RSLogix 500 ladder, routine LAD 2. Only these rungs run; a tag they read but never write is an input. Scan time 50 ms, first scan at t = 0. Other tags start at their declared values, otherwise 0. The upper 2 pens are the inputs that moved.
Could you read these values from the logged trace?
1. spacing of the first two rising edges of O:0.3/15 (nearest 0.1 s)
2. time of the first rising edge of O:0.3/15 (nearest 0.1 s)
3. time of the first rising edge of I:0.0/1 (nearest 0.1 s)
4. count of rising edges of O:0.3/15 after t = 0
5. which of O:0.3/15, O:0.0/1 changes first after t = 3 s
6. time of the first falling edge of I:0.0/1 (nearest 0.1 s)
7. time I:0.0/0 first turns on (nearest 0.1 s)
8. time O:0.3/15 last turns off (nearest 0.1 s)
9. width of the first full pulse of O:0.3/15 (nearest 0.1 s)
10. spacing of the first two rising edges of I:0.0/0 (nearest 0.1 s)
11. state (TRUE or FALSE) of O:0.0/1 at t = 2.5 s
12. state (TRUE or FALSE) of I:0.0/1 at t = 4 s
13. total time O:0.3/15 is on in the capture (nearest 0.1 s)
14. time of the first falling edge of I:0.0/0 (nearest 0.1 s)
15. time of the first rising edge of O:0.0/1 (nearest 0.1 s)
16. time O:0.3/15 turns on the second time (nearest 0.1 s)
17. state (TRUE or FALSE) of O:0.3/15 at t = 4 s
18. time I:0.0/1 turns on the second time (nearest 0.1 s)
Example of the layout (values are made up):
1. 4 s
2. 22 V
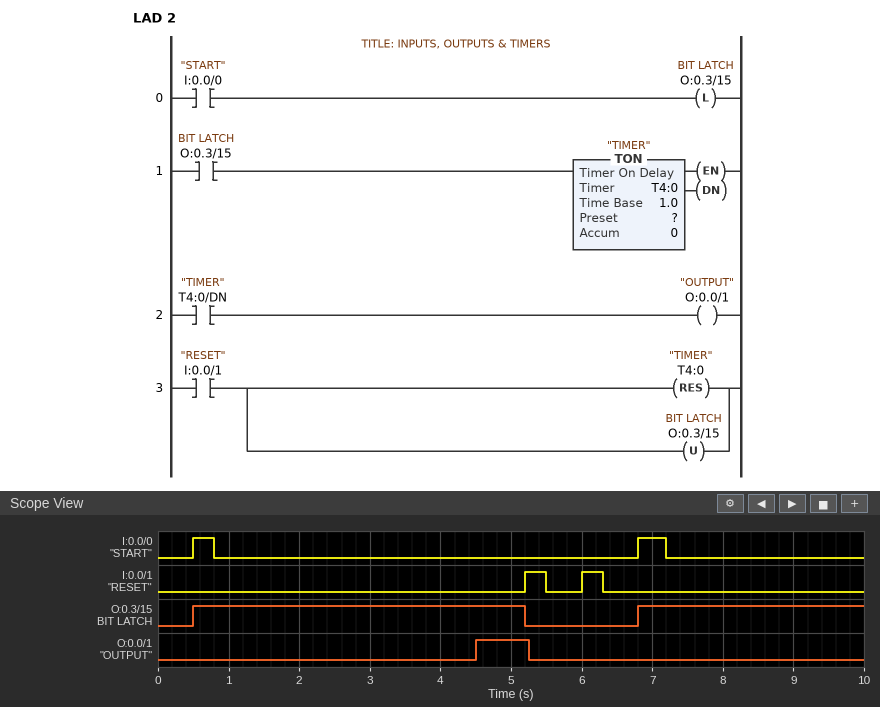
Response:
1. 6.3 s
2. 0.5 s
3. 5.2 s
4. 2
5. O:0.0/1
6. 5.5 s
7. 0.5 s
8. 5.2 s
9. 4.7 s
10. 6.3 s
11. FALSE
12. FALSE
13. 7.9 s
14. 0.8 s
15. 4.5 s
16. 6.8 s
17. TRUE
18. 6.0 s
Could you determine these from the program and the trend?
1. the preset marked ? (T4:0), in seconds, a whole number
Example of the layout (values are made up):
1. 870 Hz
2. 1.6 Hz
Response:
1. 4 s
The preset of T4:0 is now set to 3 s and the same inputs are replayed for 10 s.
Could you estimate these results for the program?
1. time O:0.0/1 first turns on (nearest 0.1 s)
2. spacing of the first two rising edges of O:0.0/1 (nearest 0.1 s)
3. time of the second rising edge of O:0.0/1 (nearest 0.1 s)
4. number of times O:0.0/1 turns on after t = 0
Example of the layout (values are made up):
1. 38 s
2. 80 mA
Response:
1. 3.5 s
2. 6.3 s
3. 9.8 s
4. 2
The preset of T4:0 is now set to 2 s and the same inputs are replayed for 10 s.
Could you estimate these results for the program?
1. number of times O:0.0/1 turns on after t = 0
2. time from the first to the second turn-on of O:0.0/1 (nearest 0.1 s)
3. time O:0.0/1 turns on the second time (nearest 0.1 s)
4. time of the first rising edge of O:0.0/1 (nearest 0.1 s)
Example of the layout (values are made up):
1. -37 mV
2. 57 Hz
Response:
1. 2
2. 6.3 s
3. 8.8 s
4. 2.5 s
